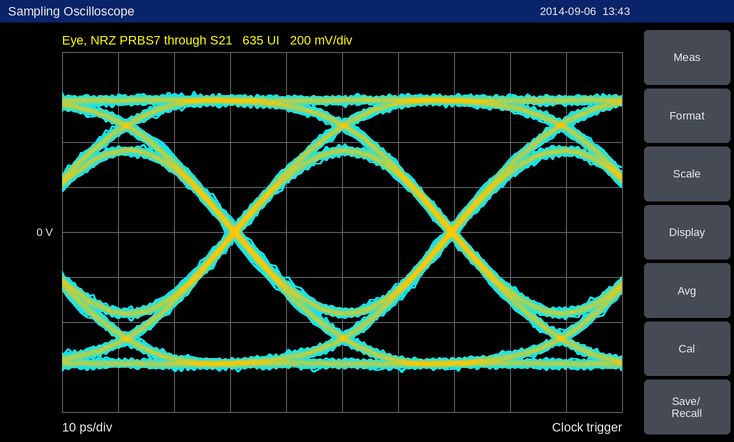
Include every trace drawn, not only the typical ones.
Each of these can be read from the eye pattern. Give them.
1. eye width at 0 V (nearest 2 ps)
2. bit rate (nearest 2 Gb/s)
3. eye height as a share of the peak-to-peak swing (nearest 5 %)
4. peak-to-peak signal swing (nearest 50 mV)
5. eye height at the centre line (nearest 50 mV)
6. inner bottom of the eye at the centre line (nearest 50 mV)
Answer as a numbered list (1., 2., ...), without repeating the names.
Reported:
1. 36 ps
2. 26 Gb/s
3. 55 %
4. 1.25 V
5. 700 mV
6. -350 mV
